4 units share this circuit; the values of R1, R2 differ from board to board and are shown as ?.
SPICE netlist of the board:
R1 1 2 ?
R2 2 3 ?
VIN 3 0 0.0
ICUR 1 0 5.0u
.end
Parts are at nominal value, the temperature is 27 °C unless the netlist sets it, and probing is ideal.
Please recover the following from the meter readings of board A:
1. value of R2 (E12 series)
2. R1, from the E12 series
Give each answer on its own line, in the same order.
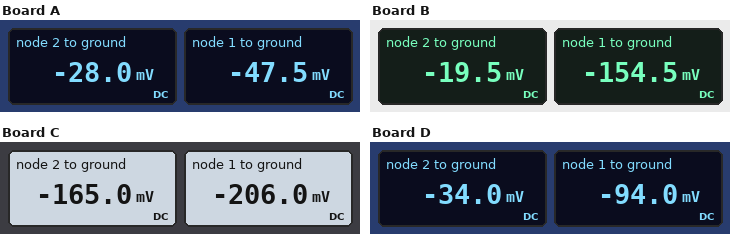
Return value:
5.6 kΩ
3.9 kΩ
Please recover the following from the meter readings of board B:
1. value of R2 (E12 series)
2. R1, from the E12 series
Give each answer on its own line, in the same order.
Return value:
3.9 kΩ
27 kΩ
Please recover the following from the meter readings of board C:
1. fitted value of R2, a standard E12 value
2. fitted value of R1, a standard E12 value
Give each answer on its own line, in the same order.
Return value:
33 kΩ
8.2 kΩ
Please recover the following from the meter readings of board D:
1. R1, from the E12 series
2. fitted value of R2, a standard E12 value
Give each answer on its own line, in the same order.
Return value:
12 kΩ
6.8 kΩ
